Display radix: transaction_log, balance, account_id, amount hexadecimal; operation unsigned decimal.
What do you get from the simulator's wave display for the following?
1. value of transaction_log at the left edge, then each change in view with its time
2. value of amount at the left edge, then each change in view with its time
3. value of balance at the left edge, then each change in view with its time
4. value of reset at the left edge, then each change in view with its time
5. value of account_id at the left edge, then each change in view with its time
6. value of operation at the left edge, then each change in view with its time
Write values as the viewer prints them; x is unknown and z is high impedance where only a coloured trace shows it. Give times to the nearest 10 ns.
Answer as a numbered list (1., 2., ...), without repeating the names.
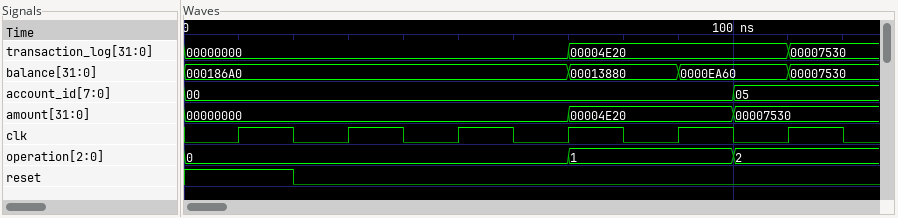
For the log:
1. 00000000, 00004E20 at 70 ns, 00007530 at 110 ns
2. 00000000, 00004E20 at 70 ns, 00007530 at 100 ns
3. 000186A0, 00013880 at 70 ns, 0000EA60 at 90 ns, 00007530 at 110 ns
4. 1, 0 at 20 ns
5. 00, 05 at 100 ns
6. 0, 1 at 70 ns, 2 at 100 ns
